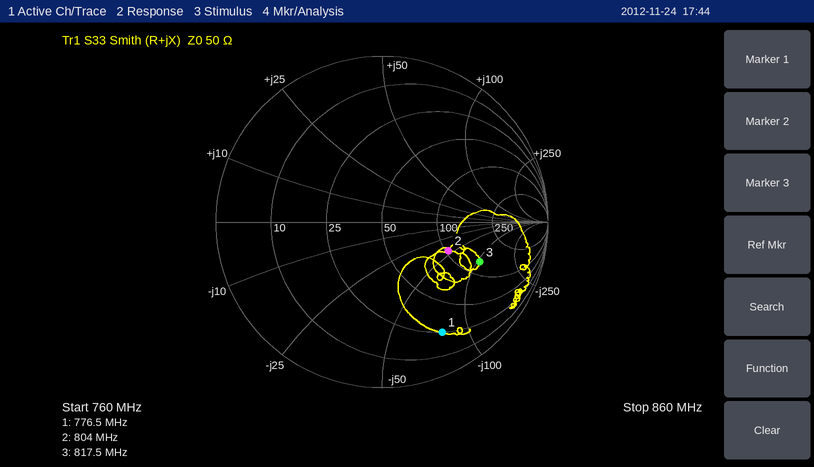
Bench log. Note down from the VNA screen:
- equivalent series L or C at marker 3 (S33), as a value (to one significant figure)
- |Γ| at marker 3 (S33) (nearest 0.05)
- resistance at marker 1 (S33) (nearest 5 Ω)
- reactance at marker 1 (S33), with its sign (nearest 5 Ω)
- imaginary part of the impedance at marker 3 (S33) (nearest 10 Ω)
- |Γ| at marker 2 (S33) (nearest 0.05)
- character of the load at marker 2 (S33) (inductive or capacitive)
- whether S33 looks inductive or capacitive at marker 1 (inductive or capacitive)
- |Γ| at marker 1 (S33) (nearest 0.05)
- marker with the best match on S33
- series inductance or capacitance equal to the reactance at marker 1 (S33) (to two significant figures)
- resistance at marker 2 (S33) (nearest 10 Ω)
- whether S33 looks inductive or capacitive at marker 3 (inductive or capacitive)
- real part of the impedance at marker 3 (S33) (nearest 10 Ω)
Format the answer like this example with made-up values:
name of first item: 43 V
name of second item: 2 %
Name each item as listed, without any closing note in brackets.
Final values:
equivalent series L or C at marker 3 (S33), as a value: 2 pF
|Γ| at marker 3 (S33): 0.65
resistance at marker 1 (S33): 25 Ω
reactance at marker 1 (S33), with its sign: -80 Ω
imaginary part of the impedance at marker 3 (S33): -110 Ω
|Γ| at marker 2 (S33): 0.45
character of the load at marker 2 (S33): capacitive
whether S33 looks inductive or capacitive at marker 1: capacitive
|Γ| at marker 1 (S33): 0.75
marker with the best match on S33: marker 2
series inductance or capacitance equal to the reactance at marker 1 (S33): 2.6 pF
resistance at marker 2 (S33): 100 Ω
whether S33 looks inductive or capacitive at marker 3: capacitive
real part of the impedance at marker 3 (S33): 130 Ω
